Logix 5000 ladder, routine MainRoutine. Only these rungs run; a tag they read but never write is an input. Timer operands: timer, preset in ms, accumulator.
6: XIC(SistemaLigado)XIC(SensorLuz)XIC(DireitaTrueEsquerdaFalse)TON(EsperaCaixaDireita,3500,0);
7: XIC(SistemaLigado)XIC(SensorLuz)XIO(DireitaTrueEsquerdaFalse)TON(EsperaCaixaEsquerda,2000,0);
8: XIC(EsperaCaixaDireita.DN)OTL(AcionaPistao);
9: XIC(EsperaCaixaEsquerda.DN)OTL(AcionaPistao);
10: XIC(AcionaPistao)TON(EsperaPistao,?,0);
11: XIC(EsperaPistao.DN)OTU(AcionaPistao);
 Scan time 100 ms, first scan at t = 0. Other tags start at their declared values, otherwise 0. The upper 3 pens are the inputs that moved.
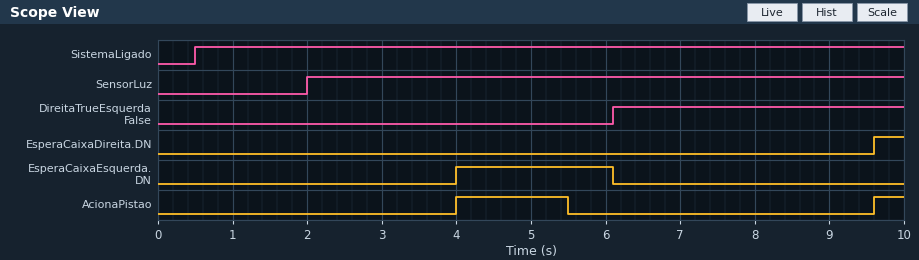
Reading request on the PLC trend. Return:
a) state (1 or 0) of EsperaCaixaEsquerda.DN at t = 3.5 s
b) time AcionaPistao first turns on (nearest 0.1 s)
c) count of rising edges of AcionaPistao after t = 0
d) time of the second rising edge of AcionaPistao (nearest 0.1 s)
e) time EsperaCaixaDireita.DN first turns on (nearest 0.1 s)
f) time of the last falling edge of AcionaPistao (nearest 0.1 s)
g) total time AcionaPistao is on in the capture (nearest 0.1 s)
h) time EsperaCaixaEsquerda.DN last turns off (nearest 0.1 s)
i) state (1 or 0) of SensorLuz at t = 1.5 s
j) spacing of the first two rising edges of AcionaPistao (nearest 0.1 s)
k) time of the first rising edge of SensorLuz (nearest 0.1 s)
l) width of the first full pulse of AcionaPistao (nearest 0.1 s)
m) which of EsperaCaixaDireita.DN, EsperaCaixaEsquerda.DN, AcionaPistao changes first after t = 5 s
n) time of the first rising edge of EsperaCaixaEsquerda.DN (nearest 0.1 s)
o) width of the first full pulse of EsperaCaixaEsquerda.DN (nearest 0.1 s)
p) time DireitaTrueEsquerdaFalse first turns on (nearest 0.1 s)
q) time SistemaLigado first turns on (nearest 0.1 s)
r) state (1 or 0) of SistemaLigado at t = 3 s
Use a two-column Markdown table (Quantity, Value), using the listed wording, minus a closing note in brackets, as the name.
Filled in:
| Quantity | Value |
|---|---|
| state (1 or 0) of EsperaCaixaEsquerda.DN at t = 3.5 s | 0 |
| time AcionaPistao first turns on | 4.0 s |
| count of rising edges of AcionaPistao after t = 0 | 2 |
| time of the second rising edge of AcionaPistao | 9.6 s |
| time EsperaCaixaDireita.DN first turns on | 9.6 s |
| time of the last falling edge of AcionaPistao | 5.5 s |
| total time AcionaPistao is on in the capture | 1.9 s |
| time EsperaCaixaEsquerda.DN last turns off | 6.1 s |
| state (1 or 0) of SensorLuz at t = 1.5 s | 0 |
| spacing of the first two rising edges of AcionaPistao | 5.6 s |
| time of the first rising edge of SensorLuz | 2.0 s |
| width of the first full pulse of AcionaPistao | 1.5 s |
| which of EsperaCaixaDireita.DN, EsperaCaixaEsquerda.DN, AcionaPistao changes first after t = 5 s | AcionaPistao |
| time of the first rising edge of EsperaCaixaEsquerda.DN | 4.0 s |
| width of the first full pulse of EsperaCaixaEsquerda.DN | 2.1 s |
| time DireitaTrueEsquerdaFalse first turns on | 6.1 s |
| time SistemaLigado first turns on | 0.5 s |
| state (1 or 0) of SistemaLigado at t = 3 s | 1 |
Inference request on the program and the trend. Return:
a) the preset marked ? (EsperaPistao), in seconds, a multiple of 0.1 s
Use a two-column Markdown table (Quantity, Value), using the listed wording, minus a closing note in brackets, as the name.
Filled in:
| Quantity | Value |
|---|---|
| the preset marked ? (EsperaPistao), in seconds, a multiple of 0.1 s | 1.5 s |
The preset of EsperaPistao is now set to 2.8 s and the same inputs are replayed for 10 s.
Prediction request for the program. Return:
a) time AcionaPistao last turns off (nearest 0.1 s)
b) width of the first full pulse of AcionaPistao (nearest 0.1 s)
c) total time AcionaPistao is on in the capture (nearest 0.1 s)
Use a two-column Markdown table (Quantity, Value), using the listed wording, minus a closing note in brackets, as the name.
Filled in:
| Quantity | Value |
|---|---|
| time AcionaPistao last turns off | 6.8 s |
| width of the first full pulse of AcionaPistao | 2.8 s |
| total time AcionaPistao is on in the capture | 3.2 s |
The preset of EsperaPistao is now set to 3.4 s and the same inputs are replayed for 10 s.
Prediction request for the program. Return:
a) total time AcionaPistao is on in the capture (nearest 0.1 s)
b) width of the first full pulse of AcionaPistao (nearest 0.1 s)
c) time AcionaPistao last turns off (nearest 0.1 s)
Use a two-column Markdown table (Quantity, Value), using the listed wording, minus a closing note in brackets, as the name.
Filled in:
| Quantity | Value |
|---|---|
| total time AcionaPistao is on in the capture | 3.8 s |
| width of the first full pulse of AcionaPistao | 3.4 s |
| time AcionaPistao last turns off | 7.4 s |
